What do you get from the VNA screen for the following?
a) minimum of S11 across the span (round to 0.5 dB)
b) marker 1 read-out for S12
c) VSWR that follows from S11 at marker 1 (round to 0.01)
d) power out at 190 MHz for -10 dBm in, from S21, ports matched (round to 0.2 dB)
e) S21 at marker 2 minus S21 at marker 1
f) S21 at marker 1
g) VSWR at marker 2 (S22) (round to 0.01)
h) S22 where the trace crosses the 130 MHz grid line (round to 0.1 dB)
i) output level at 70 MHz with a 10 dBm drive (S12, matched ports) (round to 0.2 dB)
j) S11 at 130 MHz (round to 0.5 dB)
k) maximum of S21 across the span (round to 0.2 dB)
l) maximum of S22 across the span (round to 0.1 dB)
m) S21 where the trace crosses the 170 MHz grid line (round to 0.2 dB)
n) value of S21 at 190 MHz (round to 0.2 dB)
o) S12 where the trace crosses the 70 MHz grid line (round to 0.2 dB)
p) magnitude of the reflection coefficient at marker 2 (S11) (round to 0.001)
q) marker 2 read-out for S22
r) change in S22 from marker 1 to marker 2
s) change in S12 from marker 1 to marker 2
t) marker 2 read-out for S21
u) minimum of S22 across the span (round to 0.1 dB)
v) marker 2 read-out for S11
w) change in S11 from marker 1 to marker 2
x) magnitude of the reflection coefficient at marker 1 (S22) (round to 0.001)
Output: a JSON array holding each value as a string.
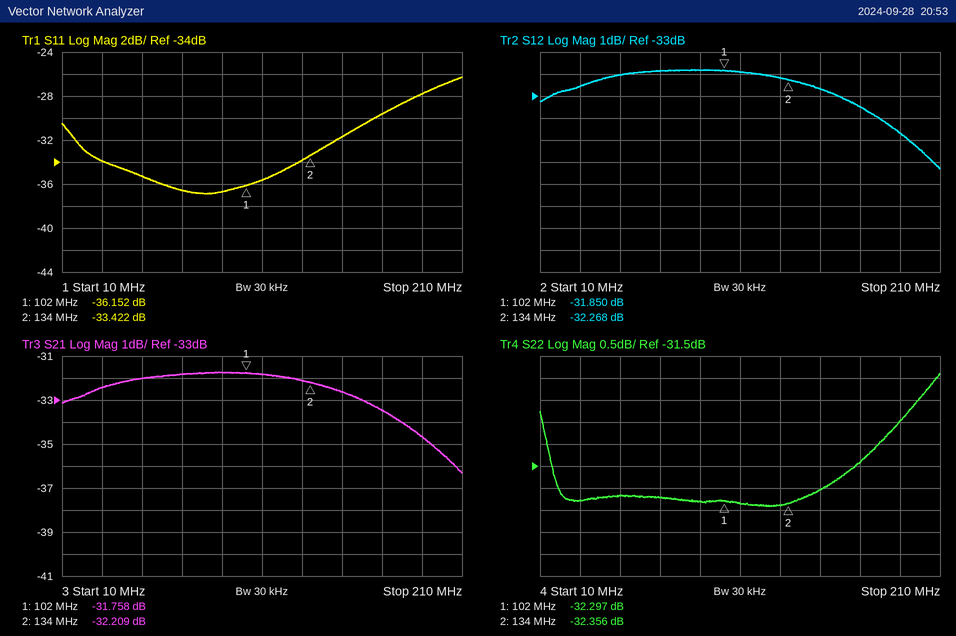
["-37.0 dB", "-31.850 dB", "1.03", "-44.6 dBm", "-0.451 dB", "-31.758 dB", "1.05", "-32.4 dB", "-21.8 dBm", "-34.0 dB", "-31.8 dB", "-29.4 dB", "-33.4 dB", "-34.6 dB", "-31.8 dB", "0.021", "-32.356 dB", "-0.059 dB", "-0.418 dB", "-32.209 dB", "-32.4 dB", "-33.422 dB", "2.730 dB", "0.024"]
